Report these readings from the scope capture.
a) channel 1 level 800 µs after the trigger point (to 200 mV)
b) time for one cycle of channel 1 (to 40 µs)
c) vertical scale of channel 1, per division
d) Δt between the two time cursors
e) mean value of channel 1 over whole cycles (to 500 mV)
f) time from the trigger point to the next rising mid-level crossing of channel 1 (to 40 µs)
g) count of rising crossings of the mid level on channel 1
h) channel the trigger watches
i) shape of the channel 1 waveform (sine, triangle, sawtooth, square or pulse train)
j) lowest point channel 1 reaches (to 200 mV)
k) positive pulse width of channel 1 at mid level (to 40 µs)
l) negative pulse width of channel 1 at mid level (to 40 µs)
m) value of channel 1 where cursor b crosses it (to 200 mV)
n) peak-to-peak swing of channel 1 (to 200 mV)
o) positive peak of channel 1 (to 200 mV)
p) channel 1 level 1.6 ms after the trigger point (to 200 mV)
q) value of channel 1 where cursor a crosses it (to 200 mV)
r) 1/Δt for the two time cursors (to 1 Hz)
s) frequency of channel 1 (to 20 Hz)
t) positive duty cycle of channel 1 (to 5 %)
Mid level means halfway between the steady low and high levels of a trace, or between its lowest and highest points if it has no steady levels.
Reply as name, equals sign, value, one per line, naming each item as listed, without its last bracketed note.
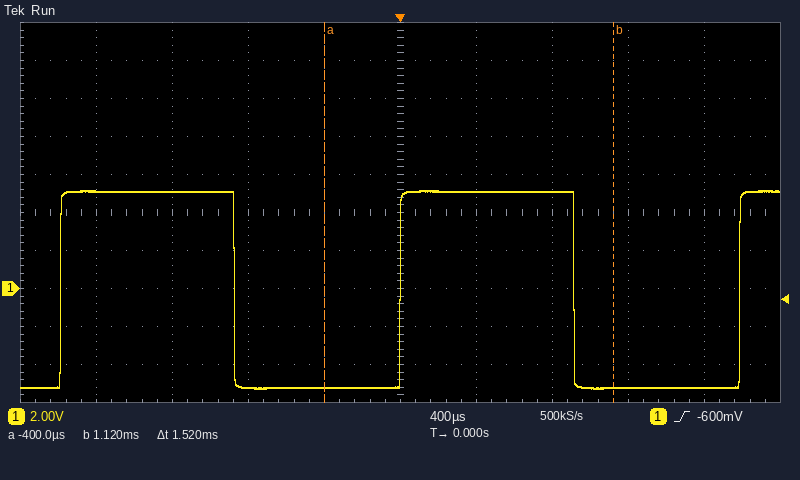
channel 1 level 800 µs after the trigger point = 5.2 V
time for one cycle of channel 1 = 1.80 ms
vertical scale of channel 1, per division = 2 V
Δt between the two time cursors = 1.52 ms
mean value of channel 1 over whole cycles = 0.0 V
time from the trigger point to the next rising mid-level crossing of channel 1 = 1.80 ms
count of rising crossings of the mid level on channel 1 = 3
channel the trigger watches = channel 1
shape of the channel 1 waveform = square
lowest point channel 1 reaches = -5.2 V
positive pulse width of channel 1 at mid level = 920 µs
negative pulse width of channel 1 at mid level = 880 µs
value of channel 1 where cursor b crosses it = -5.2 V
peak-to-peak swing of channel 1 = 10.4 V
positive peak of channel 1 = 5.2 V
channel 1 level 1.6 ms after the trigger point = -5.2 V
value of channel 1 where cursor a crosses it = -5.2 V
1/Δt for the two time cursors = 658 Hz
frequency of channel 1 = 560 Hz
positive duty cycle of channel 1 = 50 %
